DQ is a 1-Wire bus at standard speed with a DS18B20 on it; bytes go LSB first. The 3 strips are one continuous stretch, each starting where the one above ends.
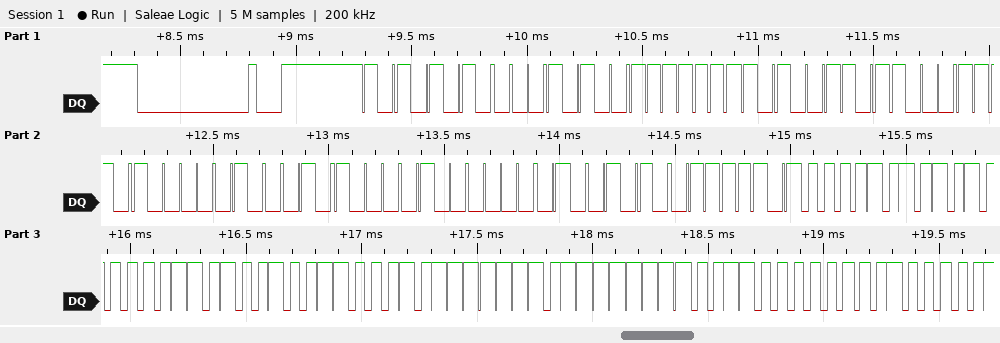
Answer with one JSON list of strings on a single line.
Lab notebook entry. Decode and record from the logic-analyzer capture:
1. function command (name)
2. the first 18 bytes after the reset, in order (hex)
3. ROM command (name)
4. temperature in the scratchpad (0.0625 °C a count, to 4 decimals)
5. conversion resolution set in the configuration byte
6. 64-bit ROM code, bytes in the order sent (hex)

["Read Scratchpad", "55 28 FF B2 71 41 14 02 52 BE 50 05 4B 46 7F FF 0C 10", "Match ROM", "85.0000 °C", "12 bits", "28 FF B2 71 41 14 02 52"]
